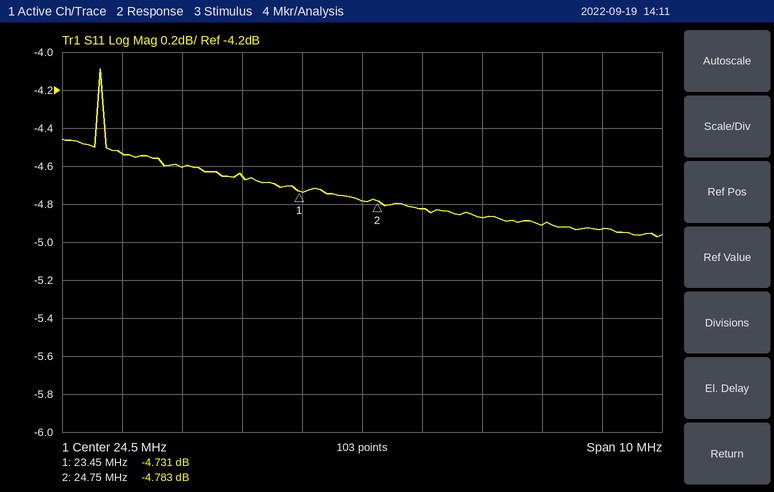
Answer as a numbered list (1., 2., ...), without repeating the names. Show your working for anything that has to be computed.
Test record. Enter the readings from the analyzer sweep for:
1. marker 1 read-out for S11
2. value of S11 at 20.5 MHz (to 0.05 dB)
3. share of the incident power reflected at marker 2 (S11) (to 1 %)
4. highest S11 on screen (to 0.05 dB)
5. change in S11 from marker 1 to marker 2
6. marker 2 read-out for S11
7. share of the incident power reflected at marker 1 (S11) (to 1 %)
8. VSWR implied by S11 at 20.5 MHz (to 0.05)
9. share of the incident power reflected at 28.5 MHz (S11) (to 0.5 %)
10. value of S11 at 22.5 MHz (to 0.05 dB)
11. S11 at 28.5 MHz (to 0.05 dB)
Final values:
1. -4.731 dB
2. -4.55 dB
3. 10^(-4.783/10) ≈ 33 %
4. -4.10 dB
5. -4.783 − (-4.731) = -0.052 dB
6. -4.783 dB
7. 10^(-4.731/10) ≈ 34 %
8. |Γ| = 10^(-4.55/20) = 0.5922; VSWR = (1 + 0.5922)/(1 − 0.5922) ≈ 3.90
9. 10^(-4.95/10) ≈ 32.0 %
10. -4.65 dB
11. -4.95 dB
